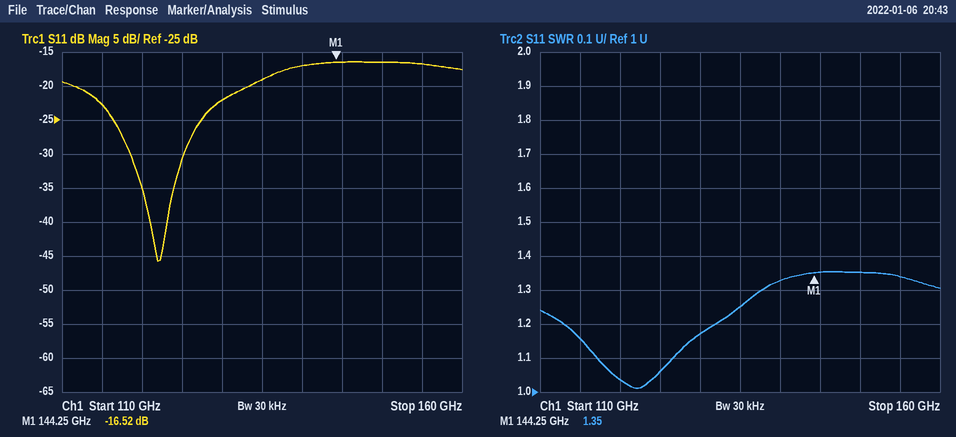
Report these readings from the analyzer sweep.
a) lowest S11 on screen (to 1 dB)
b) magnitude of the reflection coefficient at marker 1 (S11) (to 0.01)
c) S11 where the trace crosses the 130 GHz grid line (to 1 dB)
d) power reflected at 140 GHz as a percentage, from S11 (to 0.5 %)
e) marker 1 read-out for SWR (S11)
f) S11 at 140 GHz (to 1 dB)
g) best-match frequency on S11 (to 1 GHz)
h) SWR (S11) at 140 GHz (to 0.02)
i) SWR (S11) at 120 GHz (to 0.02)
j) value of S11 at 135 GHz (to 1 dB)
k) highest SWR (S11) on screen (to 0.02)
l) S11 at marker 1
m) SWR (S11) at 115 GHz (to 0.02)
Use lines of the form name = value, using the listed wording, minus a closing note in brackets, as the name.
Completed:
lowest S11 on screen = -46 dB
magnitude of the reflection coefficient at marker 1 (S11) = 0.15
S11 where the trace crosses the 130 GHz grid line = -22 dB
power reflected at 140 GHz as a percentage, from S11 = 2.0 %
marker 1 read-out for SWR = 1.35
S11 at 140 GHz = -17 dB
best-match frequency on S11 = 122 GHz
SWR (S11) at 140 GHz = 1.32
SWR (S11) at 120 GHz = 1.04
value of S11 at 135 GHz = -19 dB
highest SWR (S11) on screen = 1.36
S11 at marker 1 = -16.52 dB
SWR (S11) at 115 GHz = 1.16
